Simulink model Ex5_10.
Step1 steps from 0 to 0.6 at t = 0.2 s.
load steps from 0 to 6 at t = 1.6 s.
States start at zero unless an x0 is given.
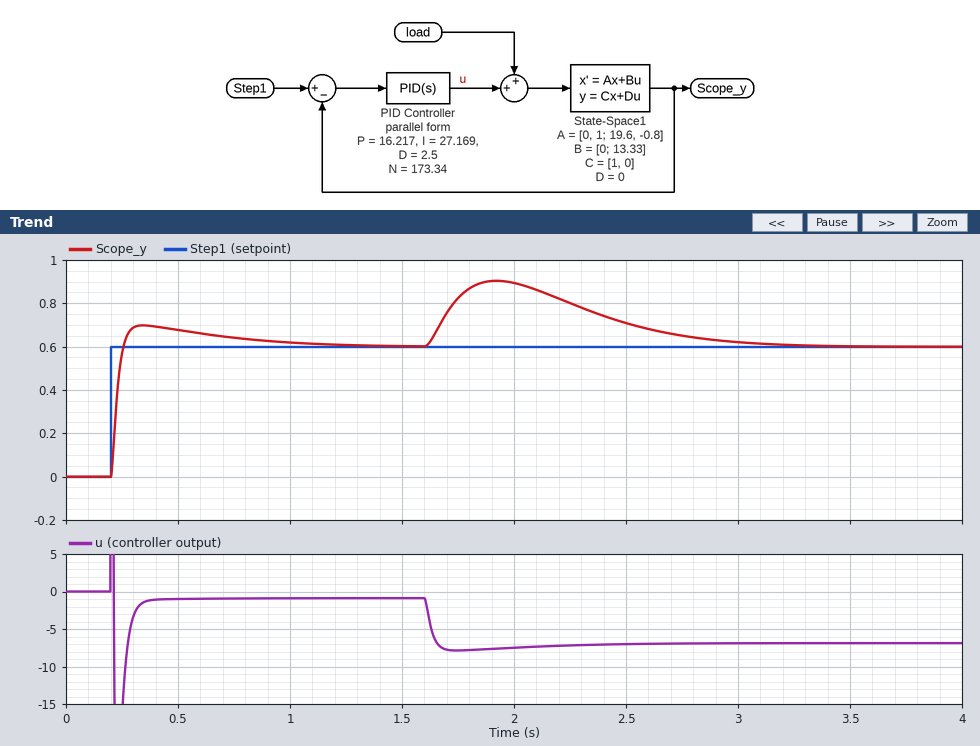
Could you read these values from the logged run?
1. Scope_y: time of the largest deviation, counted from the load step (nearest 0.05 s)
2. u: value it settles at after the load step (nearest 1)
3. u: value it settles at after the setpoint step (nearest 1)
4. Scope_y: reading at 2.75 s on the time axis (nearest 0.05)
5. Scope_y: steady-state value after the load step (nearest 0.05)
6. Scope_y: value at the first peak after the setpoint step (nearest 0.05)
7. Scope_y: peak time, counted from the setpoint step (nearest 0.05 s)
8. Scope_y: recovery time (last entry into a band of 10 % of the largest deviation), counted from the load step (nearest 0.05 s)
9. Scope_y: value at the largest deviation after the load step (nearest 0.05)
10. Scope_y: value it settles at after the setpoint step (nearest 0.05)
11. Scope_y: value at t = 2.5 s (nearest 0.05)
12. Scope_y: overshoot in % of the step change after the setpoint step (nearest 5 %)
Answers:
0.30 s
-7
-1
0.65
0.60
0.70
0.15 s
1.30 s
0.90
0.60
0.70
15 %
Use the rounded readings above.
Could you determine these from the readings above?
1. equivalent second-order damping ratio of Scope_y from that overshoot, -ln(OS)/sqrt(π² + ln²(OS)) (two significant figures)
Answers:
0.52
